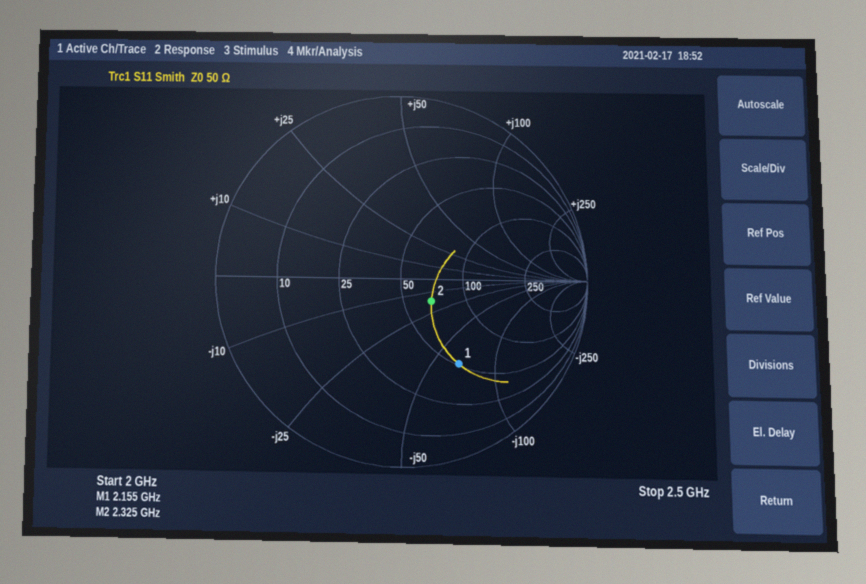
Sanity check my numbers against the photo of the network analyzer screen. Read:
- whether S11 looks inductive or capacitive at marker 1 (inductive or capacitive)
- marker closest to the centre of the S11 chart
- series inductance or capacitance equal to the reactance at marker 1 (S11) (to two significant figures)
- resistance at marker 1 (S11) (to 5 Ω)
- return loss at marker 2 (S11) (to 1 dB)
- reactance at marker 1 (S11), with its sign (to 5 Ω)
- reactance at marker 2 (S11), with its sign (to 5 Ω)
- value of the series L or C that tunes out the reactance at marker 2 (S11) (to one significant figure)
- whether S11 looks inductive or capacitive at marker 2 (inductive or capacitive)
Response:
capacitive
marker 2
1.1 pF
50 Ω
14 dB
-65 Ω
-15 Ω
1 nH
capacitive
